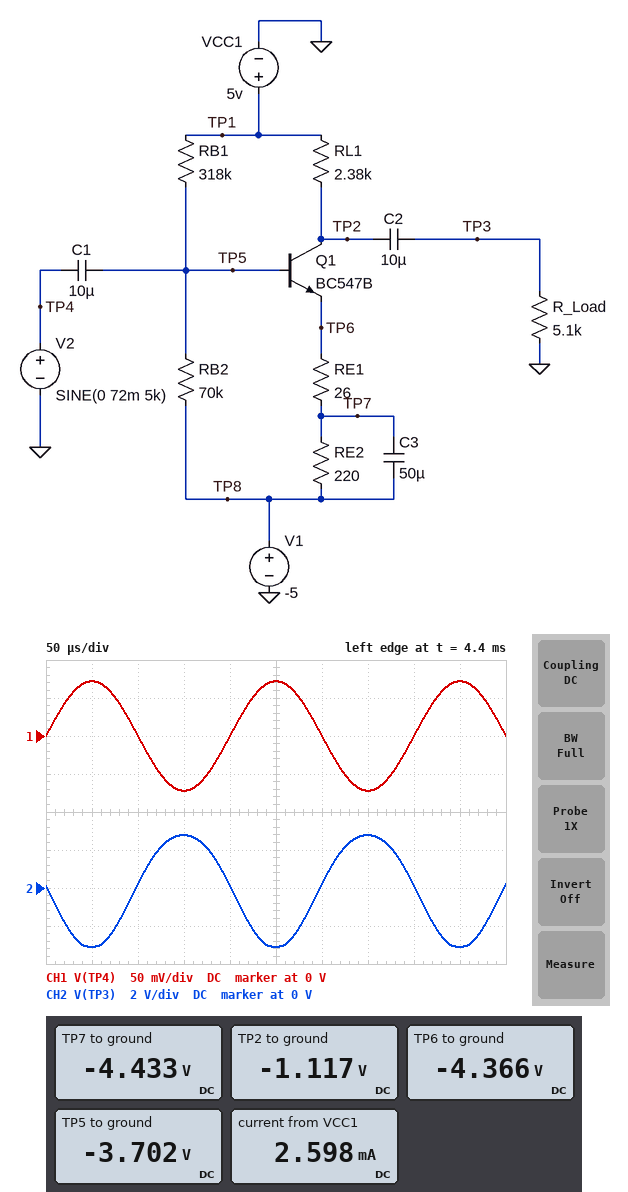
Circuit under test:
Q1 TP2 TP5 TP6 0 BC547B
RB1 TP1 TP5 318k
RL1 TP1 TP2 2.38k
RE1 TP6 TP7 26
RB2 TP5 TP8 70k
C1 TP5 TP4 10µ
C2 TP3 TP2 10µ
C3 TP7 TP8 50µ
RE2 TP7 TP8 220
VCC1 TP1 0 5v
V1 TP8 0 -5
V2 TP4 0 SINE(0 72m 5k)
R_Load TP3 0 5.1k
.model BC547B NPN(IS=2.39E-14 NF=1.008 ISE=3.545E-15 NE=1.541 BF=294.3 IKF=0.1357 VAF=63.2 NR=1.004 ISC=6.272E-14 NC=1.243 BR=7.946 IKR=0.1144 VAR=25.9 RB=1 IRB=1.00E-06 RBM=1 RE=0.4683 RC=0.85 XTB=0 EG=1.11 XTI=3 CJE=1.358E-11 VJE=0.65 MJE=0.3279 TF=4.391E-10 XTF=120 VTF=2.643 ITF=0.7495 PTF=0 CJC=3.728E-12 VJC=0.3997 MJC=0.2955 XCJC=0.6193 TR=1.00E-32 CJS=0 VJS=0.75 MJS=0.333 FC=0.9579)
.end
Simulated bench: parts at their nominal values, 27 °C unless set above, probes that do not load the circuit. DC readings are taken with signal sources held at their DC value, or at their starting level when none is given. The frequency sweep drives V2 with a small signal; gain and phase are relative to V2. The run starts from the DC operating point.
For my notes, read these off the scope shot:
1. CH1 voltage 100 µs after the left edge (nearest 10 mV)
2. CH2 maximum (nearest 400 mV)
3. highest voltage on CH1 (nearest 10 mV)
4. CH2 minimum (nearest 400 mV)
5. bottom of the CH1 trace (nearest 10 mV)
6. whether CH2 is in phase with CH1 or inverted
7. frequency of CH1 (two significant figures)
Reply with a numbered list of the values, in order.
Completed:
1. 0 V
2. 2.8 V
3. 70 mV
4. -3.2 V
5. -70 mV
6. inverted
7. 5.0 kHz
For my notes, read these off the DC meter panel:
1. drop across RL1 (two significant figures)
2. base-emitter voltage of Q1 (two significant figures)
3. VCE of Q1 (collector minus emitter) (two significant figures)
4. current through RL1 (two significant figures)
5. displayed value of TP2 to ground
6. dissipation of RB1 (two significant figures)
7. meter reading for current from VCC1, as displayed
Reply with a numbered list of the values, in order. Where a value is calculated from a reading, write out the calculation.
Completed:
1. 5 V - (-1.117 V) = 6.1 V
2. -3.702 V - (-4.366 V) = 660 mV
3. -1.117 V - (-4.366 V) = 3.2 V
4. (5 V - (-1.117 V)) / 2.38 kΩ = 2.6 mA
5. -1.117 V
6. (5 V - (-3.702 V))^2 / 318 kΩ = 240 µW
7. 2.598 mA
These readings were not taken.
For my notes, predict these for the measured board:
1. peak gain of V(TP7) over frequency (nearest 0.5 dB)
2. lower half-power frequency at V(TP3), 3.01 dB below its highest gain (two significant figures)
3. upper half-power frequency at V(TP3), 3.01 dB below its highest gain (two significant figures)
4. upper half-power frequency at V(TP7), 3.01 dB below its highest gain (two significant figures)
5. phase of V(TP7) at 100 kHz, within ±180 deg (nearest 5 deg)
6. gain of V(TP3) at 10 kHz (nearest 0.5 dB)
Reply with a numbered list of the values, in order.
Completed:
1. -1.5 dB
2. 99 Hz
3. 46 MHz
4. 100 Hz
5. -90 deg
6. 32.5 dB
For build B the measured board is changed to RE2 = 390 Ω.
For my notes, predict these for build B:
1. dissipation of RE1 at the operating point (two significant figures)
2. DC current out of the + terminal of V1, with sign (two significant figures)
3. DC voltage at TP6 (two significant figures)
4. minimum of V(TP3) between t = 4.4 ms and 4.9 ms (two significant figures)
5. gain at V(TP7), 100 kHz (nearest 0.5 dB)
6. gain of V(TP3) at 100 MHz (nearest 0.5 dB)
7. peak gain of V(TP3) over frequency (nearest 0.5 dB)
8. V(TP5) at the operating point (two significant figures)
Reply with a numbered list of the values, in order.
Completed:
1. 93 µW
2. -1.9 mA
3. -4.2 V
4. -2.9 V
5. -62.0 dB
6. 24.5 dB
7. 32.0 dB
8. -3.6 V
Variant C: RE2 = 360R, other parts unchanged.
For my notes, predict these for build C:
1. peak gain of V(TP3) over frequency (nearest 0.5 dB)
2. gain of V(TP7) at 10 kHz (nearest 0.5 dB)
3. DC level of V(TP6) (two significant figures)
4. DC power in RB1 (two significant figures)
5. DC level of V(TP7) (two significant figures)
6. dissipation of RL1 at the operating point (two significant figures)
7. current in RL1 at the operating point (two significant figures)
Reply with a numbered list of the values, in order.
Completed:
1. 32.0 dB
2. -42.0 dB
3. -4.2 V
4. 230 µW
5. -4.3 V
6. 9.3 mW
7. 2.0 mA
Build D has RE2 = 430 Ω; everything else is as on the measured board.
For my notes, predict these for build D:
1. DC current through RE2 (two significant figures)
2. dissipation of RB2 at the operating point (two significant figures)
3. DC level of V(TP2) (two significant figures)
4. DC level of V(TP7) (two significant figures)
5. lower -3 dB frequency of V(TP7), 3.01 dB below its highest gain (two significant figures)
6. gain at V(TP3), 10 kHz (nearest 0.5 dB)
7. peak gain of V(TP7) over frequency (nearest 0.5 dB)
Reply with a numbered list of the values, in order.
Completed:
1. 1.8 mA
2. 31 µW
3. 770 mV
4. -4.2 V
5. 390 mHz
6. 31.5 dB
7. -1.0 dB
